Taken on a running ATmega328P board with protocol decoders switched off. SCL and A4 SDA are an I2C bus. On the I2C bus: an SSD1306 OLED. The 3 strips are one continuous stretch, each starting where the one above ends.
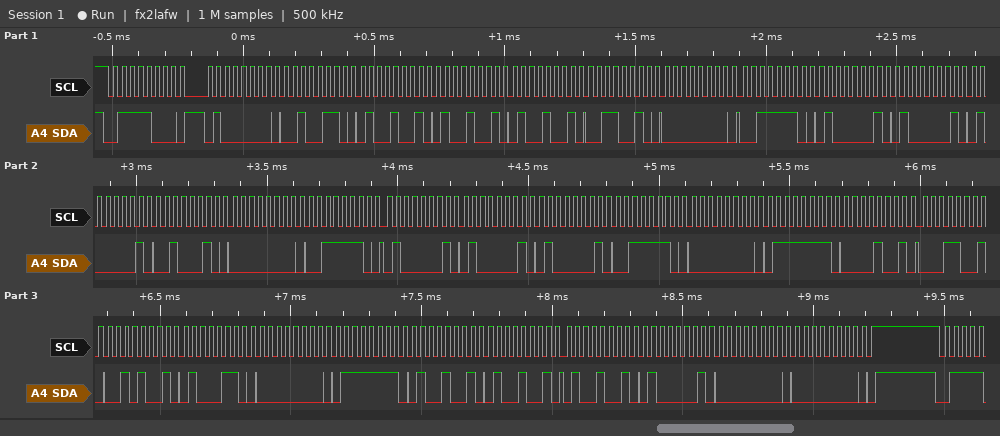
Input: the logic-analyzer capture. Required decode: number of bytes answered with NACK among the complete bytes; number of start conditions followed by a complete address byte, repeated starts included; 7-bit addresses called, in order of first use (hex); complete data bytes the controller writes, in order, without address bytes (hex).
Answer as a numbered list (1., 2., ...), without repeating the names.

1. 0
2. 1
3. 0x3C
4. 40 26 49 49 49 32 00 3E 41 41 41 22 00 3E 41 41 41 3E 00 7F 09 19 29 46 00 7F 49 49 49 41 00 00
